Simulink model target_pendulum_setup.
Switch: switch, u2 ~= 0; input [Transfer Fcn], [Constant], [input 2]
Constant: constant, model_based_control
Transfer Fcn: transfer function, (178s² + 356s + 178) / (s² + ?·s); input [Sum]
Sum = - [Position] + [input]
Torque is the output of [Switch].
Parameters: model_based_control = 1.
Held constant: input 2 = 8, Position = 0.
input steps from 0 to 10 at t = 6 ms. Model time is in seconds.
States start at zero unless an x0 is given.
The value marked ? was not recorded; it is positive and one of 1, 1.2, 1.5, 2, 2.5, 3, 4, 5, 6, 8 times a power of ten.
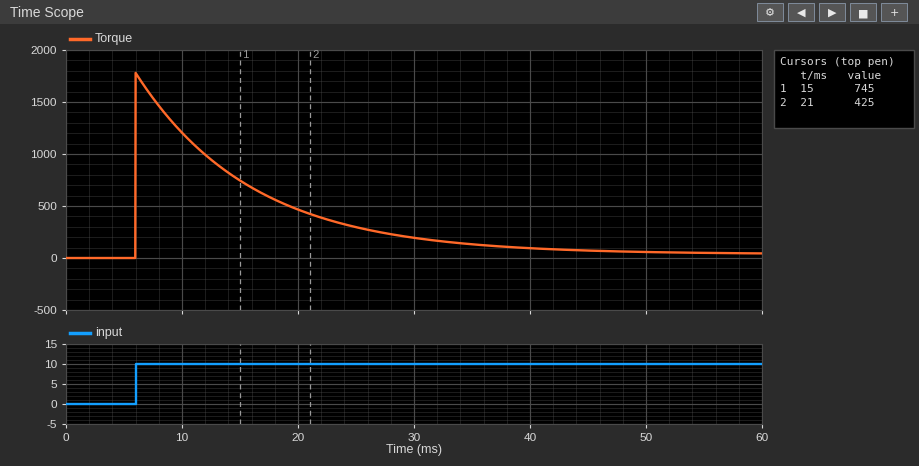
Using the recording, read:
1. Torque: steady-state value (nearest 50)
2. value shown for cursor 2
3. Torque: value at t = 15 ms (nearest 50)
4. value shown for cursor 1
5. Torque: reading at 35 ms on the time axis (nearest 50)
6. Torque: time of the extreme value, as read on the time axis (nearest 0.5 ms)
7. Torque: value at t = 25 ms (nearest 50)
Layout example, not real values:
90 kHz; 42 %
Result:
50; 425; 750; 745; 150; 6.0 ms; 300
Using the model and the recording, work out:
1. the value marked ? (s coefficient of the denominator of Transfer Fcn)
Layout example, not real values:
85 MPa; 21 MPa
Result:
100
